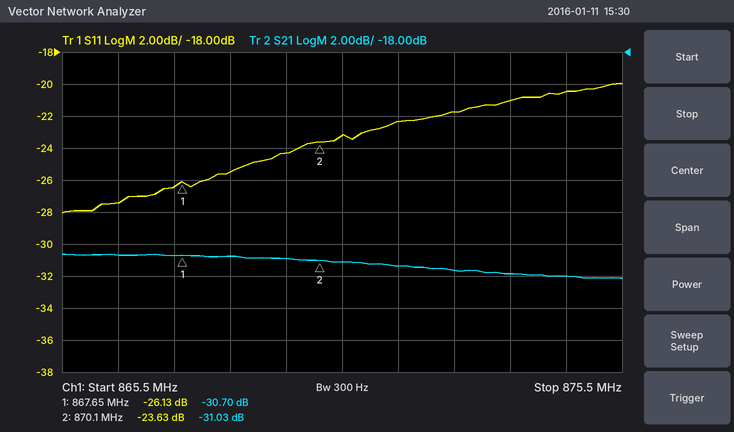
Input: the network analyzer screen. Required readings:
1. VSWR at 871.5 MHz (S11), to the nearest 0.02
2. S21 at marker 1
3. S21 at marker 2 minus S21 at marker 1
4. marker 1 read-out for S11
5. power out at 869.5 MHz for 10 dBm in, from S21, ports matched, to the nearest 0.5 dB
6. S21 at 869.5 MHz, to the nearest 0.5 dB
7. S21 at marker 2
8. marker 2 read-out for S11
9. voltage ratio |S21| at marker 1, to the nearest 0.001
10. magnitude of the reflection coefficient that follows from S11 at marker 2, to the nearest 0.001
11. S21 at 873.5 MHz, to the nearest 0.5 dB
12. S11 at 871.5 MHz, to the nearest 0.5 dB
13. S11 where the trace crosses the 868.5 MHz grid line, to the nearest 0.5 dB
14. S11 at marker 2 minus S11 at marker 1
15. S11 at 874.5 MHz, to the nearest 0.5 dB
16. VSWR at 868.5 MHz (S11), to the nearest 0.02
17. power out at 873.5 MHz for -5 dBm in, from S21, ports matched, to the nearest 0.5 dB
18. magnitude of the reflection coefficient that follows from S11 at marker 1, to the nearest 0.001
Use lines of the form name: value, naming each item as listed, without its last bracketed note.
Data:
VSWR at 871.5 MHz (S11), to the nearest 0.02: 1.16
S21 at marker 1: -30.70 dB
S21 at marker 2 minus S21 at marker 1: -0.33 dB
marker 1 read-out for S11: -26.13 dB
power out at 869.5 MHz for 10 dBm in, from S21, ports matched, to the nearest 0.5 dB: -21.0 dBm
S21 at 869.5 MHz, to the nearest 0.5 dB: -31.0 dB
S21 at marker 2: -31.03 dB
marker 2 read-out for S11: -23.63 dB
voltage ratio |S21| at marker 1, to the nearest 0.001: 0.029
magnitude of the reflection coefficient that follows from S11 at marker 2, to the nearest 0.001: 0.066
S21 at 873.5 MHz, to the nearest 0.5 dB: -32.0 dB
S11 at 871.5 MHz, to the nearest 0.5 dB: -22.5 dB
S11 where the trace crosses the 868.5 MHz grid line, to the nearest 0.5 dB: -25.5 dB
S11 at marker 2 minus S11 at marker 1: 2.50 dB
S11 at 874.5 MHz, to the nearest 0.5 dB: -20.5 dB
VSWR at 868.5 MHz (S11), to the nearest 0.02: 1.12
power out at 873.5 MHz for -5 dBm in, from S21, ports matched, to the nearest 0.5 dB: -37.0 dBm
magnitude of the reflection coefficient that follows from S11 at marker 1, to the nearest 0.001: 0.049
